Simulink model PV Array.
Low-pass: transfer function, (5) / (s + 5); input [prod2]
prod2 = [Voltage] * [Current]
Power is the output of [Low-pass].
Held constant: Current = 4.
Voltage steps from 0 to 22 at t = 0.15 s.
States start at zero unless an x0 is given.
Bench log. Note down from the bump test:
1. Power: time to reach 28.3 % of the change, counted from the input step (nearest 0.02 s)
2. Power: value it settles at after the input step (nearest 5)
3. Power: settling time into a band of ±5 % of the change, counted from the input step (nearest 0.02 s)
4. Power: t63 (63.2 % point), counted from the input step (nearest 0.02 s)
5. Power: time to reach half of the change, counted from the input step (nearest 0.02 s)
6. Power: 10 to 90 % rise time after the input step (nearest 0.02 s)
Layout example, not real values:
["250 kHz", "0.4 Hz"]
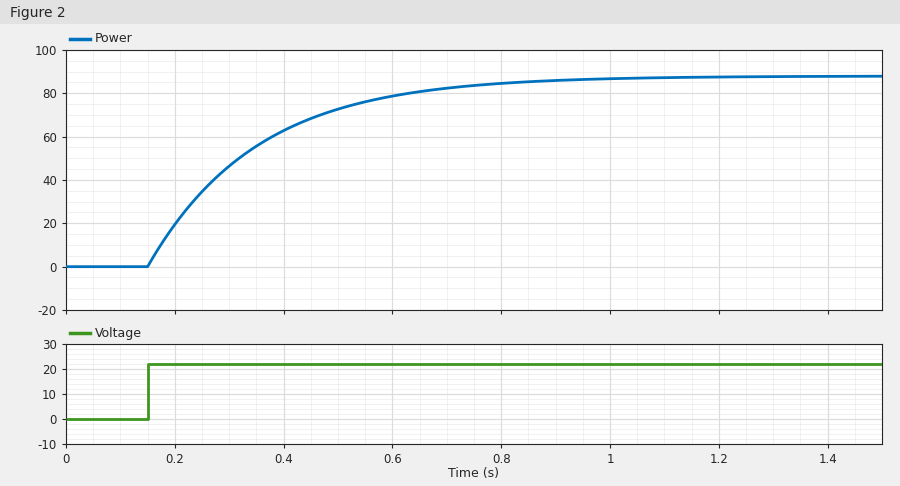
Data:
["0.06 s", "90", "0.60 s", "0.20 s", "0.14 s", "0.44 s"]
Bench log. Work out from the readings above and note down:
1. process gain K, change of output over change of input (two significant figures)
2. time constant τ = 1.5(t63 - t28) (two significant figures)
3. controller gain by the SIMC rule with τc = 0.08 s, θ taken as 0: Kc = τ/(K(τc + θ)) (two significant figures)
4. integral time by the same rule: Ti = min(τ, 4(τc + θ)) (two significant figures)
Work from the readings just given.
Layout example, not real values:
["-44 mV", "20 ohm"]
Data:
["4.1", "0.21 s", "0.64", "0.21 s"]
